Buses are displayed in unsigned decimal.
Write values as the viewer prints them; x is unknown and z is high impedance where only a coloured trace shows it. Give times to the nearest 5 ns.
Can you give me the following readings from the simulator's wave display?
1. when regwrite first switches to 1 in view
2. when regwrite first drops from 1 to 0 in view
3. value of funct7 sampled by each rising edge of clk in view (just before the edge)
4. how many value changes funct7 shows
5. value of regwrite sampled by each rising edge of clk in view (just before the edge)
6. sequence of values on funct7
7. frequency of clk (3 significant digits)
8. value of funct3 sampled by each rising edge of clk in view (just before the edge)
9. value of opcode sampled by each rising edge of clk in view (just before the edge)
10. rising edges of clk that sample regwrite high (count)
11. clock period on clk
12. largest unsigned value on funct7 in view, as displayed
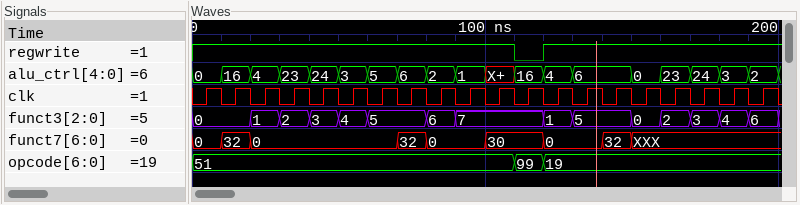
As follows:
120 ns
110 ns
0, 32, 0, 0, 0, 0, 0, 32, 0, 0, 30, 30, 0, 0, 32, XXX, XXX, XXX, XXX, XXX
8
1 1 1 1 1 1 1 1 1 1 1 0 1 1 1 1 1 1 1 1
0, 32, 0, 32, 0, 30, 0, 32, XXX
100 MHz
0, 0, 1, 2, 3, 4, 5, 5, 6, 7, 7, 7, 1, 5, 5, 0, 2, 3, 4, 6
51, 51, 51, 51, 51, 51, 51, 51, 51, 51, 51, 99, 19, 19, 19, 19, 19, 19, 19, 19
19
10 ns
32
